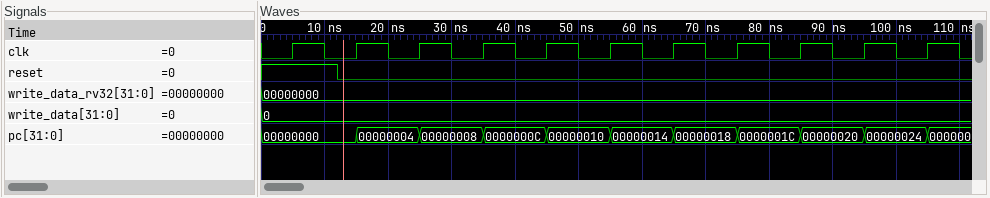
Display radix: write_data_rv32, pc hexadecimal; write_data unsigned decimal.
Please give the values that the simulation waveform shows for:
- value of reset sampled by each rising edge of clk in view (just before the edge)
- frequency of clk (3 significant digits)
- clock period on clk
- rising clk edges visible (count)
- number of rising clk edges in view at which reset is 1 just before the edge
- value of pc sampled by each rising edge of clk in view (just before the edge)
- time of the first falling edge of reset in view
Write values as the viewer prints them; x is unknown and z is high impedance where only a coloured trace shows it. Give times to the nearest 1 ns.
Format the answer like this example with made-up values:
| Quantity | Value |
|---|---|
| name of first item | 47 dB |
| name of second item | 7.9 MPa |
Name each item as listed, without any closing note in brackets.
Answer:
| Quantity | Value |
|---|---|
| value of reset sampled by each rising edge of clk in view | 1 0 0 0 0 0 0 0 0 0 0 |
| frequency of clk | 100 MHz |
| clock period on clk | 10 ns |
| rising clk edges visible | 11 |
| number of rising clk edges in view at which reset is 1 just before the edge | 1 |
| value of pc sampled by each rising edge of clk in view | 00000000, 00000000, 00000004, 00000008, 0000000C, 00000010, 00000014, 00000018, 0000001C, 00000020, 00000024 |
| time of the first falling edge of reset in view | 12 ns |
